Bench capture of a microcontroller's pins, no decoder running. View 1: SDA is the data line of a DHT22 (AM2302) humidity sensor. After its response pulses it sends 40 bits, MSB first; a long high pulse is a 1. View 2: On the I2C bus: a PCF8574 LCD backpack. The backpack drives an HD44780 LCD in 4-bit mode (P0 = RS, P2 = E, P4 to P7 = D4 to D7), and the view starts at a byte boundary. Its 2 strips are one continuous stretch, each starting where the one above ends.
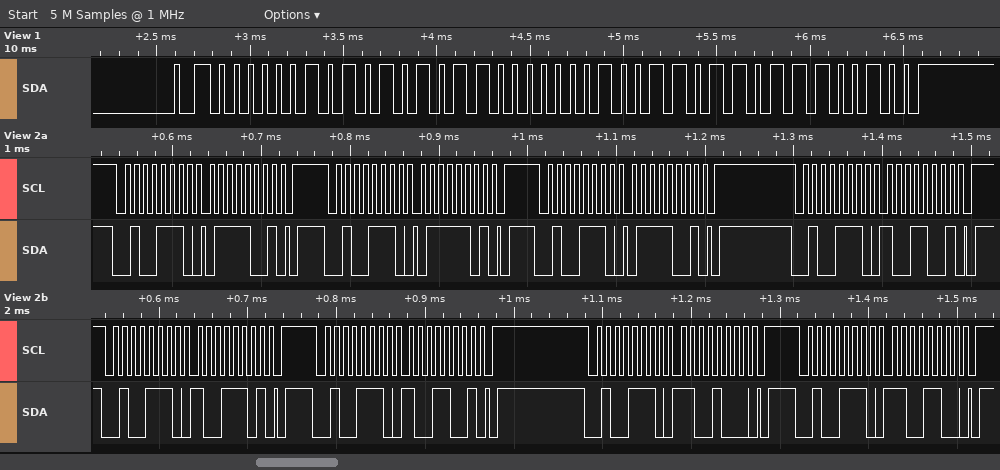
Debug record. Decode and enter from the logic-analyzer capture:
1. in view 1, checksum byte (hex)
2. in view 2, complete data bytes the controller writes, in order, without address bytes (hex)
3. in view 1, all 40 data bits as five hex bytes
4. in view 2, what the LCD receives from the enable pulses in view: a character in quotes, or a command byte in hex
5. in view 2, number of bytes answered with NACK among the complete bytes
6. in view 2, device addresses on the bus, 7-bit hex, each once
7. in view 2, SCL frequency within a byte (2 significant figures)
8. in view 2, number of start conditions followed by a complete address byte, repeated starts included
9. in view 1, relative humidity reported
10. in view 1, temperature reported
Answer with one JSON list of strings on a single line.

["0xE4", "79 7D 79 99 9D 99 C8 CC", "02 AB 01 36 E4", "'y'", "0", "0x27", "100 kHz", "8", "68.3 %", "31.0 °C"]
